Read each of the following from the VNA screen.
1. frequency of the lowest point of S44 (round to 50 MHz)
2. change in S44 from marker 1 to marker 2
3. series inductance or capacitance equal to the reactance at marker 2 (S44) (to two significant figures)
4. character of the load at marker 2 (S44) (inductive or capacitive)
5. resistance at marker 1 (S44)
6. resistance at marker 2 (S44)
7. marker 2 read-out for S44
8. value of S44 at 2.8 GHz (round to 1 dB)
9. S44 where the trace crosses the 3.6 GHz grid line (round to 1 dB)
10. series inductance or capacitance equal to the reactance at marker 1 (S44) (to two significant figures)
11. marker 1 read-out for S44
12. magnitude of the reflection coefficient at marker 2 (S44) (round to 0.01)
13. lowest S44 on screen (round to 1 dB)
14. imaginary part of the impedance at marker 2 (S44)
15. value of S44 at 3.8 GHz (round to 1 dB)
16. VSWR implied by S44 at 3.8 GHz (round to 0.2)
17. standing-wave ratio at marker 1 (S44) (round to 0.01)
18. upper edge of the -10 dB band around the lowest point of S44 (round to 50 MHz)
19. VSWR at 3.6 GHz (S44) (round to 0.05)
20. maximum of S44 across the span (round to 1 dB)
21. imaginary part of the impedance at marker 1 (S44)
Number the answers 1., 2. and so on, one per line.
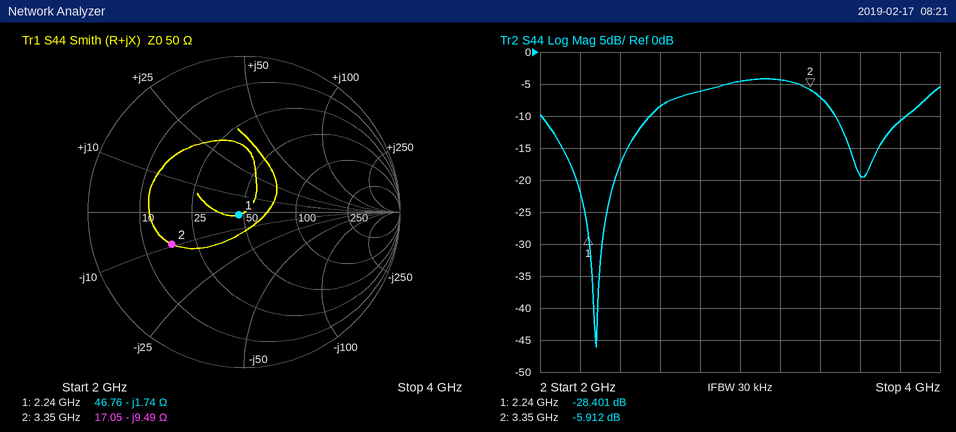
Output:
1. 2.30 GHz
2. 22.489 dB
3. 5.0 pF
4. capacitive
5. 46.76 Ω
6. 17.05 Ω
7. -5.912 dB
8. -6 dB
9. -19 dB
10. 41 pF
11. -28.401 dB
12. 0.51
13. -46 dB
14. -9.49 Ω
15. -11 dB
16. 1.8
17. 1.08
18. 2.55 GHz
19. 1.25
20. -4 dB
21. -1.74 Ω
